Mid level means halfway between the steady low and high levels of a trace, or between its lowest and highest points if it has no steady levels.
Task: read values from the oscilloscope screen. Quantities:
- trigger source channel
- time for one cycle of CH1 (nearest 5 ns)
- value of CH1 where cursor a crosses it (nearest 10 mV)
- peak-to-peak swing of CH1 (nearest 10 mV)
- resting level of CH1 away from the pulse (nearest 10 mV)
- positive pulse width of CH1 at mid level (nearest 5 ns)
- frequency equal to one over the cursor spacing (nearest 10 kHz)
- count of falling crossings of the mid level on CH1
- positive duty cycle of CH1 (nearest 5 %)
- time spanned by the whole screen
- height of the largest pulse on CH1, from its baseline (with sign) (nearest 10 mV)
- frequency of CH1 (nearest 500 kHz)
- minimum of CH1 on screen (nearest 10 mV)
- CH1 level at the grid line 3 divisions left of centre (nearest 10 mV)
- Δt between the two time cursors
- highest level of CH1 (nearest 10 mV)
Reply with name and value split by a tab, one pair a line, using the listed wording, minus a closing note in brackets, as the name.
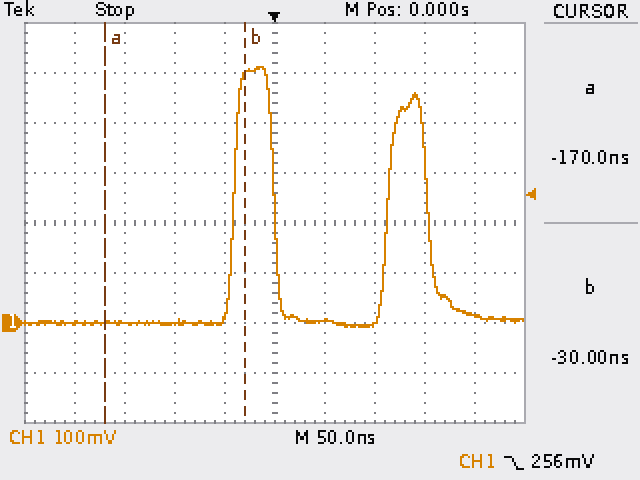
trigger source channel	CH1
time for one cycle of CH1	155 ns
value of CH1 where cursor a crosses it	0 mV
peak-to-peak swing of CH1	520 mV
resting level of CH1 away from the pulse	0 mV
positive pulse width of CH1 at mid level	40 ns
frequency equal to one over the cursor spacing	7.14 MHz
count of falling crossings of the mid level on CH1	2
positive duty cycle of CH1	25 %
time spanned by the whole screen	500 ns
height of the largest pulse on CH1, from its baseline (with sign)	+510 mV
frequency of CH1	6.5 MHz
minimum of CH1 on screen	-10 mV
CH1 level at the grid line 3 divisions left of centre	0 mV
Δt between the two time cursors	140 ns
highest level of CH1	510 mV
